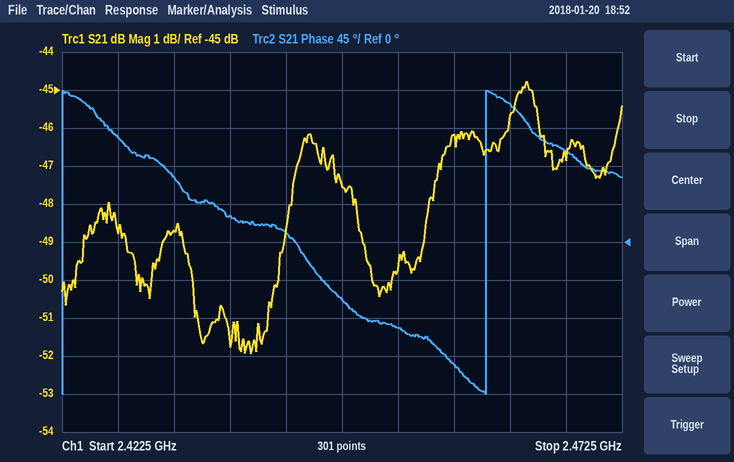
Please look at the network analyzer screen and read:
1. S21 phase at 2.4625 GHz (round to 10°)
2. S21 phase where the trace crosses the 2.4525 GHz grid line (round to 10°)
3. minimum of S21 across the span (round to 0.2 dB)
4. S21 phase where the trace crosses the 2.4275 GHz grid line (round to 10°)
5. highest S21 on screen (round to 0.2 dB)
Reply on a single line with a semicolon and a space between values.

160°; -100°; -52.0 dB; 120°; -44.8 dB
